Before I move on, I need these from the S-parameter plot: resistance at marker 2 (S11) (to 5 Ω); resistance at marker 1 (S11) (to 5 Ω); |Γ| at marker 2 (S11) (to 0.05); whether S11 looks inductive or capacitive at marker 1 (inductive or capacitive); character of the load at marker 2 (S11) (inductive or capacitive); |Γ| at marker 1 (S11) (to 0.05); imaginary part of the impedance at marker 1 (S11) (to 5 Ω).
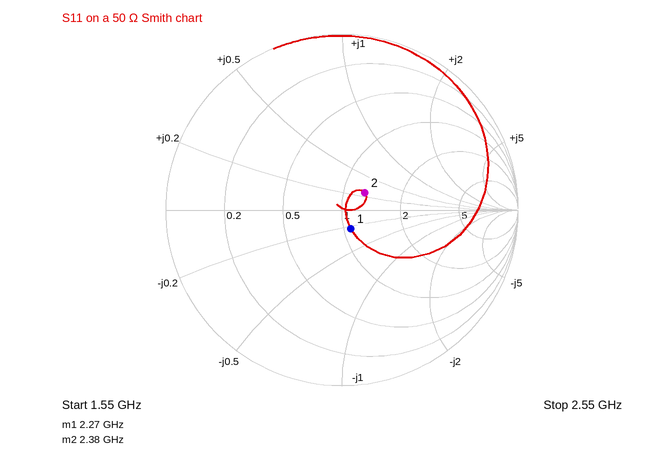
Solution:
65 Ω
55 Ω
0.15
capacitive
inductive
0.10
-10 Ω
